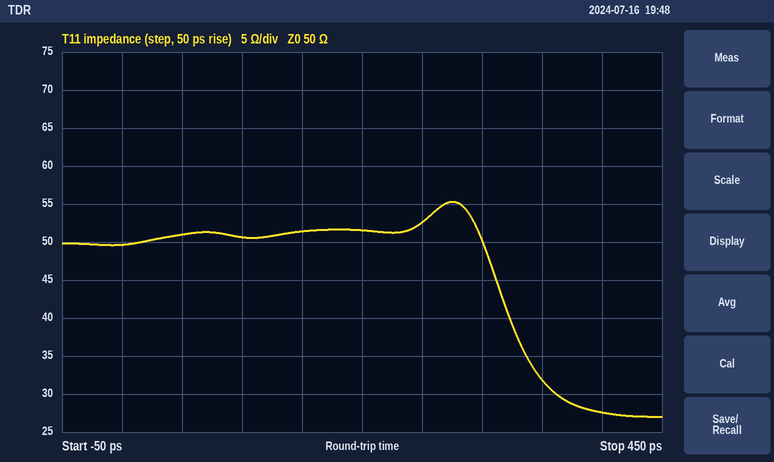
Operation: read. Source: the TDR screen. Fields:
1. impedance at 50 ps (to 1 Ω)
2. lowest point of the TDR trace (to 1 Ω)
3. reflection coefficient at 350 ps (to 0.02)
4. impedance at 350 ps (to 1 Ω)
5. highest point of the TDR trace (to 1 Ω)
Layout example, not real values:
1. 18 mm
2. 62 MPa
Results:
1. 51 Ω
2. 27 Ω
3. -0.22
4. 32 Ω
5. 55 Ω
